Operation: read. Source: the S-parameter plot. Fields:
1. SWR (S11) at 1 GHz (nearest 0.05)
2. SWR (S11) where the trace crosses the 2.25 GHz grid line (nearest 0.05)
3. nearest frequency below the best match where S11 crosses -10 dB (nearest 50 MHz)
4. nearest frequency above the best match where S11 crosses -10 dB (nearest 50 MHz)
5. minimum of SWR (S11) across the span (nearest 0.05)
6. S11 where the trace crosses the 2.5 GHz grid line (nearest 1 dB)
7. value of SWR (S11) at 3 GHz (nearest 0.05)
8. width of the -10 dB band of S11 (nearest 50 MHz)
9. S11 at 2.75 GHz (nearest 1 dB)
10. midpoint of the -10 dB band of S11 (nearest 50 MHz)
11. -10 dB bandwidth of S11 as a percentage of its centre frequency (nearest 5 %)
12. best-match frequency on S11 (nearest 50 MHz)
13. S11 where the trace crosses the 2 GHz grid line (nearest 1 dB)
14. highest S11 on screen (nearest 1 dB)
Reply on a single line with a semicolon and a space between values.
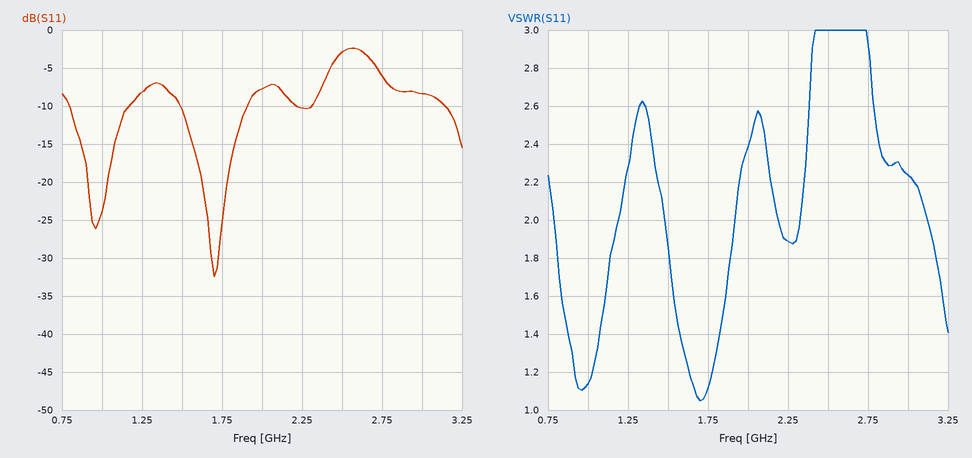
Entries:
1.15; 1.90; 1.50 GHz; 1.90 GHz; 1.05; -3 dB; 2.25; 400 MHz; -6 dB; 1.70 GHz; 25 %; 1.70 GHz; -8 dB; -2 dB
